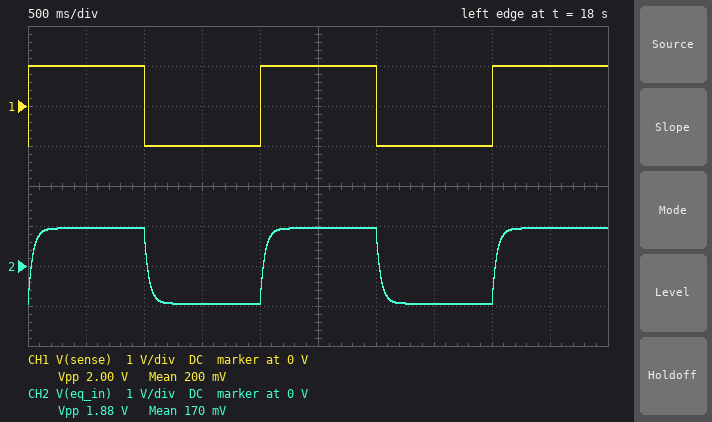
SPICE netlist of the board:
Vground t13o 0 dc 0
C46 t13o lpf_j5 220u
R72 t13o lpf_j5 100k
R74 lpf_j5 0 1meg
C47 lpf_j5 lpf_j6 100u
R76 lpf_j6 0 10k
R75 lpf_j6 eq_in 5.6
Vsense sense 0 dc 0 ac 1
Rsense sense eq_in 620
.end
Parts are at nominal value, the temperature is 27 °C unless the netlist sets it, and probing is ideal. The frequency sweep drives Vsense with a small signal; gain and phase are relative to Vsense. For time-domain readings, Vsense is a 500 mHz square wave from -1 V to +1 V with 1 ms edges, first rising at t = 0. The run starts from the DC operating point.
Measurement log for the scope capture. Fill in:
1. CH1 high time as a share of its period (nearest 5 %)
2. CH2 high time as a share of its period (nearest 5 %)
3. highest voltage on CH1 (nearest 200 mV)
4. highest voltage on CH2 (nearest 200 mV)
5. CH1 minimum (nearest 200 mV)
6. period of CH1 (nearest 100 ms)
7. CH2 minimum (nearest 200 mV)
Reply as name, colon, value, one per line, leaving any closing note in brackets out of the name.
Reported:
CH1 high time as a share of its period: 50 %
CH2 high time as a share of its period: 50 %
highest voltage on CH1: 1.0 V
highest voltage on CH2: 1.0 V
CH1 minimum: -1.0 V
period of CH1: 2.0 s
CH2 minimum: -1.0 V
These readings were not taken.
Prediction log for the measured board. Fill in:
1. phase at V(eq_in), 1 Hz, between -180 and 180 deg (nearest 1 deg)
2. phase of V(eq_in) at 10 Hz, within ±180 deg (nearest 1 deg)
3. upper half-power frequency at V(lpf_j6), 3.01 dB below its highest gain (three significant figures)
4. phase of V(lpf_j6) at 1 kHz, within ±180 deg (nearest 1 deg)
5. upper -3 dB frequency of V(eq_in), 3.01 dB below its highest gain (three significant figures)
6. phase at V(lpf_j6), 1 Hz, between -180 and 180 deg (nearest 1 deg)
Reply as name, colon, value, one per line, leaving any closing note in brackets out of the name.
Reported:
phase at V(eq_in), 1 Hz, between -180 and 180 deg: -14 deg
phase of V(eq_in) at 10 Hz, within ±180 deg: -67 deg
upper half-power frequency at V(lpf_j6), 3.01 dB below its highest gain: 3.93 Hz
phase of V(lpf_j6) at 1 kHz, within ±180 deg: -90 deg
upper -3 dB frequency of V(eq_in), 3.01 dB below its highest gain: 3.93 Hz
phase at V(lpf_j6), 1 Hz, between -180 and 180 deg: -14 deg
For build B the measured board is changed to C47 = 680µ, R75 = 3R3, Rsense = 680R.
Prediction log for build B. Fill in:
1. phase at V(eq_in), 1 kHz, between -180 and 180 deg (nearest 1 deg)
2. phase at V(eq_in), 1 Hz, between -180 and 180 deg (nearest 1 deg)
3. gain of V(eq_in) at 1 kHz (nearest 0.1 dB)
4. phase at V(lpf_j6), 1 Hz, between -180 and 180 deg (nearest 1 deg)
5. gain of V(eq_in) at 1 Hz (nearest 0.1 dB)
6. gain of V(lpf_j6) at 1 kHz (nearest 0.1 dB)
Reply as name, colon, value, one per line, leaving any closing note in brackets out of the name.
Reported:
phase at V(eq_in), 1 kHz, between -180 and 180 deg: -16 deg
phase at V(eq_in), 1 Hz, between -180 and 180 deg: -33 deg
gain of V(eq_in) at 1 kHz: -46.0 dB
phase at V(lpf_j6), 1 Hz, between -180 and 180 deg: -34 deg
gain of V(eq_in) at 1 Hz: -2.2 dB
gain of V(lpf_j6) at 1 kHz: -57.1 dB
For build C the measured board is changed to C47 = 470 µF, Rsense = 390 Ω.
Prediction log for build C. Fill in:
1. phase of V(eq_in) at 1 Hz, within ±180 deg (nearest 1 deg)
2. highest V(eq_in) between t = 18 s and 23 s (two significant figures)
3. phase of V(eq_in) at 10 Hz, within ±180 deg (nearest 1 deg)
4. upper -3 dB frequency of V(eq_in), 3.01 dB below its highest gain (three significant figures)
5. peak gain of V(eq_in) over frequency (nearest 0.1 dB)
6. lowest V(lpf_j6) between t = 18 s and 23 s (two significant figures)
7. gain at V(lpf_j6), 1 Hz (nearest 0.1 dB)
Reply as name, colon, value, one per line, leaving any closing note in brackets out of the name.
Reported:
phase of V(eq_in) at 1 Hz, within ±180 deg: -19 deg
highest V(eq_in) between t = 18 s and 23 s: 960 mV
phase of V(eq_in) at 10 Hz, within ±180 deg: -71 deg
upper -3 dB frequency of V(eq_in), 3.01 dB below its highest gain: 2.79 Hz
peak gain of V(eq_in) over frequency: -0.3 dB
lowest V(lpf_j6) between t = 18 s and 23 s: -960 mV
gain at V(lpf_j6), 1 Hz: -0.9 dB
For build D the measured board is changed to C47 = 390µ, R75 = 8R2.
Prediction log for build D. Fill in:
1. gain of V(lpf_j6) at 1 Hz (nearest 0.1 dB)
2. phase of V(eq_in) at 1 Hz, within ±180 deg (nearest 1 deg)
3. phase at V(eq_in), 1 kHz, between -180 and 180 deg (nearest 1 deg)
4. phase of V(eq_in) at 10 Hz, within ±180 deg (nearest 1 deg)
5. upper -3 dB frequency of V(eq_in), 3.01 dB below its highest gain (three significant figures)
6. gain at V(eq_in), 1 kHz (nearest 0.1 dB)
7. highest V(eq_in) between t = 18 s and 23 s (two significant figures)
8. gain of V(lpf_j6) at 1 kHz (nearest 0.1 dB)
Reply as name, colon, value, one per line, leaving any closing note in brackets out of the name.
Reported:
gain of V(lpf_j6) at 1 Hz: -1.6 dB
phase of V(eq_in) at 1 Hz, within ±180 deg: -27 deg
phase at V(eq_in), 1 kHz, between -180 and 180 deg: -8 deg
phase of V(eq_in) at 10 Hz, within ±180 deg: -75 deg
upper -3 dB frequency of V(eq_in), 3.01 dB below its highest gain: 1.91 Hz
gain at V(eq_in), 1 kHz: -37.6 dB
highest V(eq_in) between t = 18 s and 23 s: 940 mV
gain of V(lpf_j6) at 1 kHz: -54.9 dB
